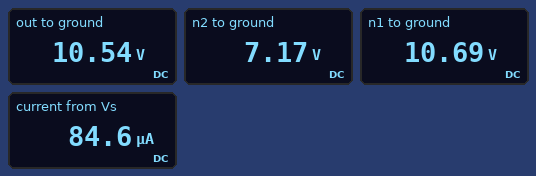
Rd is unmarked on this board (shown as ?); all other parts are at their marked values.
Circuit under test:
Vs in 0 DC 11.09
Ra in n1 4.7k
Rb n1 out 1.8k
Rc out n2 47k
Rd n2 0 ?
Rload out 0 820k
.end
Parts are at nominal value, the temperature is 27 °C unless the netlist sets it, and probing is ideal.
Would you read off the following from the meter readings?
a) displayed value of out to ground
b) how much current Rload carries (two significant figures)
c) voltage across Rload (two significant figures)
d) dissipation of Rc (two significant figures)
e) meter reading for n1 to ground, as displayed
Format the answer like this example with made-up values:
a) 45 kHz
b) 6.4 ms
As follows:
a) 10.54 V
b) 13 µA
c) 11 V
d) 240 µW
e) 10.69 V
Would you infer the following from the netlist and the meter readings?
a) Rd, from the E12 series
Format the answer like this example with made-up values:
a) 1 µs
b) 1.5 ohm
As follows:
a) 100 kΩ
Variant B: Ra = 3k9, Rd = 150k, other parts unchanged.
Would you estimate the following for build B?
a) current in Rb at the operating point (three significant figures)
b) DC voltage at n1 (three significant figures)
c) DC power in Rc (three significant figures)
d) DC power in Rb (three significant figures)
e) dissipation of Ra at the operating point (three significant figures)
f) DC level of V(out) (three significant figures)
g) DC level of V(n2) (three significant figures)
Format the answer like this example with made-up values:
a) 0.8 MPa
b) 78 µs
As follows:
a) 67.4 µA
b) 10.8 V
c) 139 µW
d) 8.18 µW
e) 17.7 µW
f) 10.7 V
g) 8.15 V
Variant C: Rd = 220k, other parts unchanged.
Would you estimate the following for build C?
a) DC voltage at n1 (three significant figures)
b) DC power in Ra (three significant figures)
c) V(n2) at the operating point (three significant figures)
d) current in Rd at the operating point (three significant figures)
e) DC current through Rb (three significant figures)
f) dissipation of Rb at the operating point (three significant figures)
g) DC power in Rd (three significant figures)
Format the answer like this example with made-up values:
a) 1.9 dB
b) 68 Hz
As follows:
a) 10.8 V
b) 13.4 µW
c) 8.85 V
d) 40.2 µA
e) 53.3 µA
f) 5.12 µW
g) 356 µW
